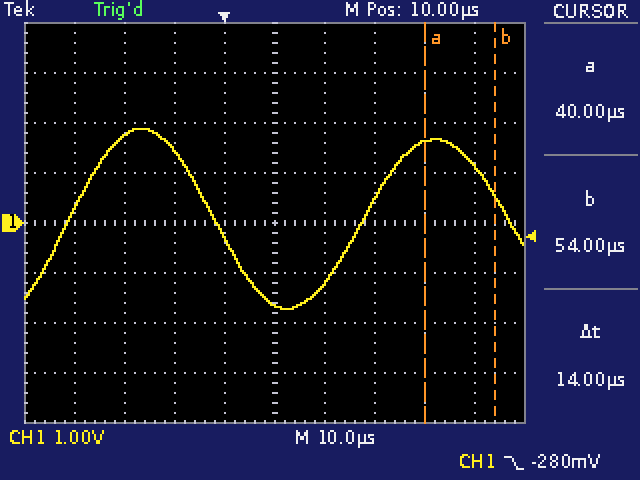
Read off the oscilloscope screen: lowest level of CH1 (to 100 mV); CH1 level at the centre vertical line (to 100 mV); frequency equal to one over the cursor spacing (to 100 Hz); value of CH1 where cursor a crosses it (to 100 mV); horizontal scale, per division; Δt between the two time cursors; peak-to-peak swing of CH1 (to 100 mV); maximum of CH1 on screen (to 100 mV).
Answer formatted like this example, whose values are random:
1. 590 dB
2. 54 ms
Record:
1. -1.7 V
2. -1.6 V
3. 71.4 kHz
4. 1.6 V
5. 10 µs
6. 14 µs
7. 3.6 V
8. 1.9 V
